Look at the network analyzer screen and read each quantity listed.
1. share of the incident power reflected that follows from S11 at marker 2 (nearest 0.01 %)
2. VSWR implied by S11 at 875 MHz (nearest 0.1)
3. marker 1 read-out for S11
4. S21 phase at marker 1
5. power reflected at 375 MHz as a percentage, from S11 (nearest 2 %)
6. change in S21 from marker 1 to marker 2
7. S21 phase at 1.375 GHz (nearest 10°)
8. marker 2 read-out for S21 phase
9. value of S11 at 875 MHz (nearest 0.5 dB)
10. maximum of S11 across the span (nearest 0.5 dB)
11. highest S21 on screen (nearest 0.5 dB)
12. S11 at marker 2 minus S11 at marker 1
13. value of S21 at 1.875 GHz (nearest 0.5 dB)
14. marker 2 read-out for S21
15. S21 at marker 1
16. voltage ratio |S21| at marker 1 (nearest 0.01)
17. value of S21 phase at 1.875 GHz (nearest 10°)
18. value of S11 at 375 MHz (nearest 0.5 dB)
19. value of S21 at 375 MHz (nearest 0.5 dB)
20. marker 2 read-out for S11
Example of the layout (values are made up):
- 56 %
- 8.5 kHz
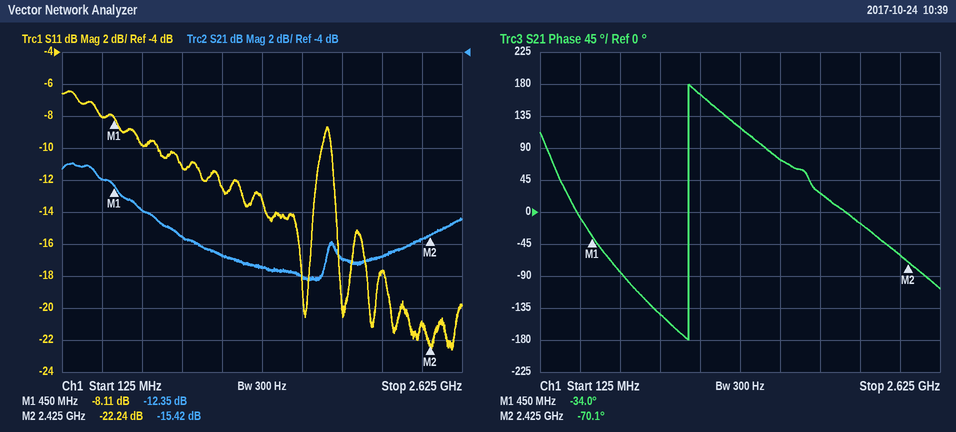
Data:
- 0.60 %
- 1.8
- -8.11 dB
- -34.0°
- 16 %
- -3.07 dB
- 120°
- -70.1°
- -11.0 dB
- -6.5 dB
- -11.0 dB
- -14.13 dB
- -17.0 dB
- -15.42 dB
- -12.35 dB
- 0.24
- 30°
- -8.0 dB
- -12.0 dB
- -22.24 dB
